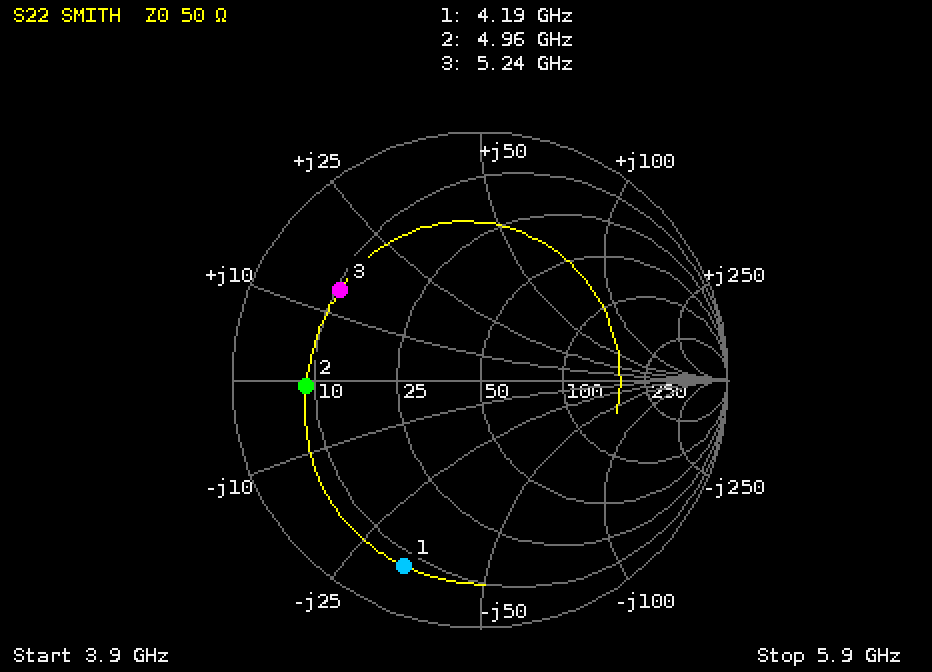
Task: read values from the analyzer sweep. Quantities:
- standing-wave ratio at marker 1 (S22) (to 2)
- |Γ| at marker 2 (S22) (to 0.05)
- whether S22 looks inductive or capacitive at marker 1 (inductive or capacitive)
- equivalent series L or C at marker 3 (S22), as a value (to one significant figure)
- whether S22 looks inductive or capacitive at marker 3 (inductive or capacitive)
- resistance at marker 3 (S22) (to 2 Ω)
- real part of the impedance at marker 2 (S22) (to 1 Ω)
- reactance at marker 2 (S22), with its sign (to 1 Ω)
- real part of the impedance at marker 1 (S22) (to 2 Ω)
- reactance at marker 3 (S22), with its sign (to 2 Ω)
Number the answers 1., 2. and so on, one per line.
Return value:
1. 10
2. 0.70
3. capacitive
4. 400 pH
5. inductive
6. 10 Ω
7. 9 Ω
8. -1 Ω
9. 8 Ω
10. +14 Ω
